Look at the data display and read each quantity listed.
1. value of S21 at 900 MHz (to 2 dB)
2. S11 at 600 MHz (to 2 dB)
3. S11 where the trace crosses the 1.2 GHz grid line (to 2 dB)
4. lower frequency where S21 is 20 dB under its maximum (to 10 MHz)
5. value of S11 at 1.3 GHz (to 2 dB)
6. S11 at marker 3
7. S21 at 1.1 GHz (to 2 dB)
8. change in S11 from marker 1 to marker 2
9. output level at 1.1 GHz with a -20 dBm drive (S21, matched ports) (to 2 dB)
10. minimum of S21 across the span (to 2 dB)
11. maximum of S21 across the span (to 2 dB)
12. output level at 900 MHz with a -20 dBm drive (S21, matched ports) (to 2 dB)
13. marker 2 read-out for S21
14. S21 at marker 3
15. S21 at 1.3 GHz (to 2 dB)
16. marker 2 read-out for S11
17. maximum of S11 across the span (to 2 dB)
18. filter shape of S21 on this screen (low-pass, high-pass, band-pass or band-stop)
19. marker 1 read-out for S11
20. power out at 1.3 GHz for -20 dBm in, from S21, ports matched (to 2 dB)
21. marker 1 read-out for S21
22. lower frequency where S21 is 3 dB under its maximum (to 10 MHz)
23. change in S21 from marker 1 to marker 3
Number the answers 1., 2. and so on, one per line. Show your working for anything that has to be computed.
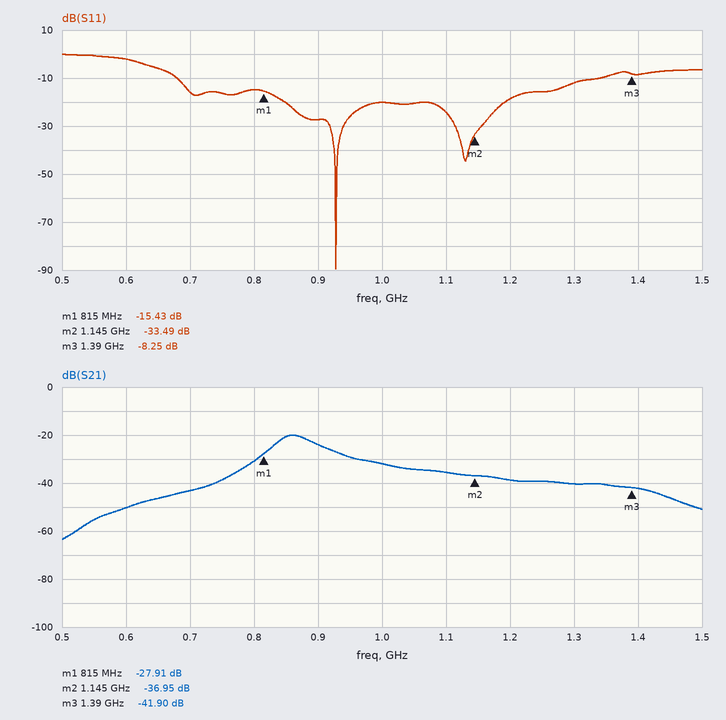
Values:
1. -24 dB
2. -2 dB
3. -18 dB
4. 740 MHz
5. -12 dB
6. -8.25 dB
7. -36 dB
8. -33.49 − (-15.43) = -18.06 dB
9. -20 dBm + (-36 dB) = -56 dBm
10. -64 dB
11. -20 dB
12. -20 dBm + (-24 dB) = -44 dBm
13. -36.95 dB
14. -41.90 dB
15. -40 dB
16. -33.49 dB
17. 0 dB
18. band-pass
19. -15.43 dB
20. -20 dBm + (-40 dB) = -60 dBm
21. -27.91 dB
22. 840 MHz
23. -41.9 − (-27.91) = -13.99 dB
